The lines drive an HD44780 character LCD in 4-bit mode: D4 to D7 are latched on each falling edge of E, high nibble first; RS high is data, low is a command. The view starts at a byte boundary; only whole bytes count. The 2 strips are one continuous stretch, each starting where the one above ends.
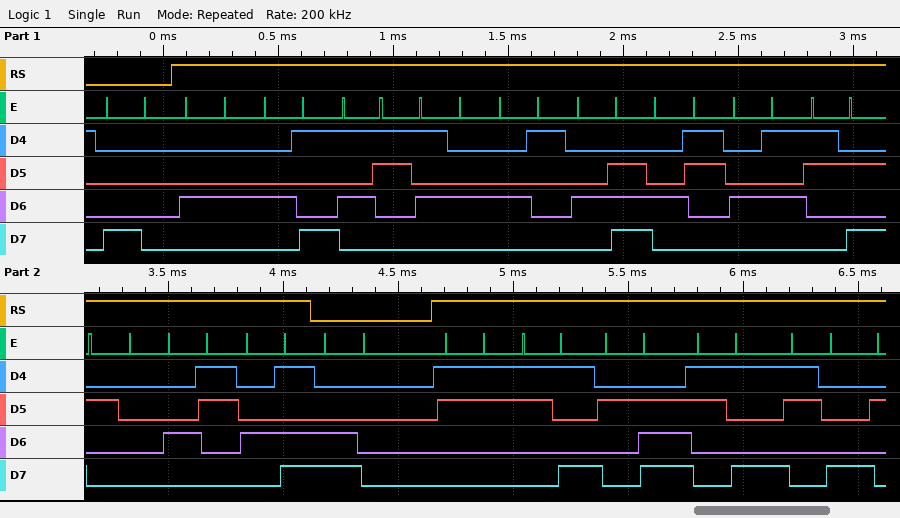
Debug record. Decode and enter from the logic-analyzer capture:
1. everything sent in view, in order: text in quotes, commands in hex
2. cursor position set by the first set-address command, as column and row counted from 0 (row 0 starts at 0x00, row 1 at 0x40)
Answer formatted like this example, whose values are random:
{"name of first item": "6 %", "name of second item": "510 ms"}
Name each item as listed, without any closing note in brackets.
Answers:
{"everything sent in view, in order: text in quotes, commands in hex": "0x80 \"DISTANCE: CM\" 0xC0 \"39.98\"", "cursor position set by the first set-address command, as column and row counted from 0": "column 0, row 0"}
